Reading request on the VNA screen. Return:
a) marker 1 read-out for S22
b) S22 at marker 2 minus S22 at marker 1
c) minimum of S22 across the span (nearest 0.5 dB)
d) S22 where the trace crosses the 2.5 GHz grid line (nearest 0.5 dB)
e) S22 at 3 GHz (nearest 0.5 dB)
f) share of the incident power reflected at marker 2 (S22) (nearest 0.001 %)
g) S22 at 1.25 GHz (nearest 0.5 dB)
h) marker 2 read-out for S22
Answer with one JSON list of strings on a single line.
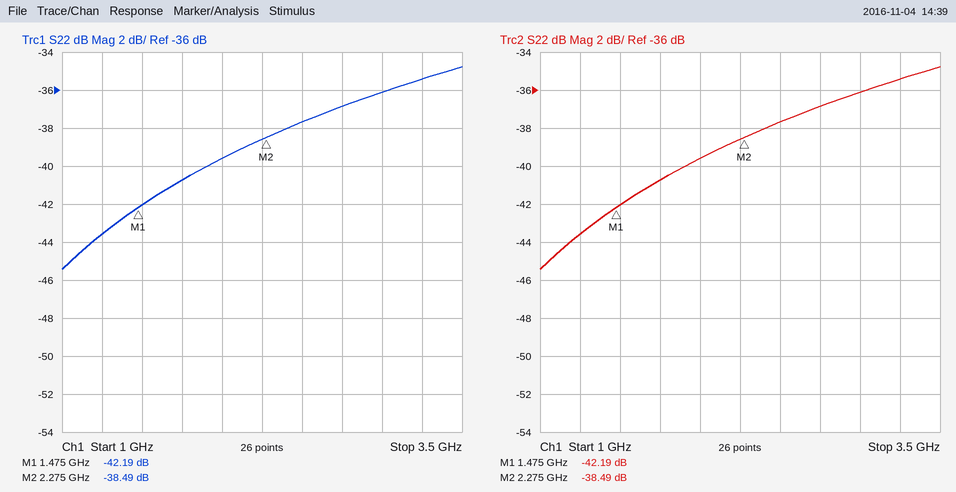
["-42.19 dB", "3.70 dB", "-45.5 dB", "-37.5 dB", "-36.0 dB", "0.014 %", "-43.5 dB", "-38.49 dB"]
